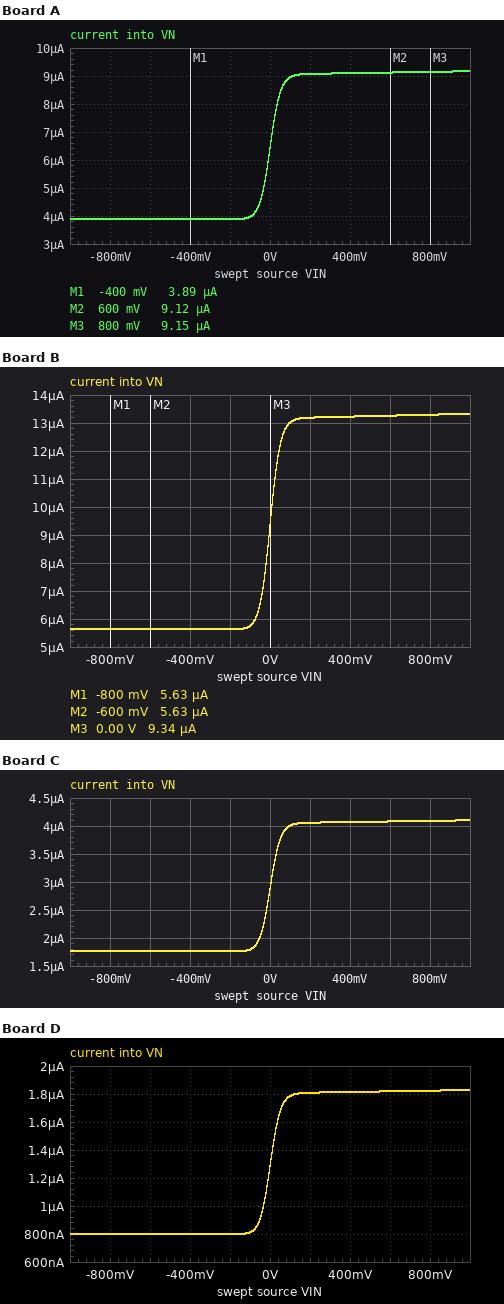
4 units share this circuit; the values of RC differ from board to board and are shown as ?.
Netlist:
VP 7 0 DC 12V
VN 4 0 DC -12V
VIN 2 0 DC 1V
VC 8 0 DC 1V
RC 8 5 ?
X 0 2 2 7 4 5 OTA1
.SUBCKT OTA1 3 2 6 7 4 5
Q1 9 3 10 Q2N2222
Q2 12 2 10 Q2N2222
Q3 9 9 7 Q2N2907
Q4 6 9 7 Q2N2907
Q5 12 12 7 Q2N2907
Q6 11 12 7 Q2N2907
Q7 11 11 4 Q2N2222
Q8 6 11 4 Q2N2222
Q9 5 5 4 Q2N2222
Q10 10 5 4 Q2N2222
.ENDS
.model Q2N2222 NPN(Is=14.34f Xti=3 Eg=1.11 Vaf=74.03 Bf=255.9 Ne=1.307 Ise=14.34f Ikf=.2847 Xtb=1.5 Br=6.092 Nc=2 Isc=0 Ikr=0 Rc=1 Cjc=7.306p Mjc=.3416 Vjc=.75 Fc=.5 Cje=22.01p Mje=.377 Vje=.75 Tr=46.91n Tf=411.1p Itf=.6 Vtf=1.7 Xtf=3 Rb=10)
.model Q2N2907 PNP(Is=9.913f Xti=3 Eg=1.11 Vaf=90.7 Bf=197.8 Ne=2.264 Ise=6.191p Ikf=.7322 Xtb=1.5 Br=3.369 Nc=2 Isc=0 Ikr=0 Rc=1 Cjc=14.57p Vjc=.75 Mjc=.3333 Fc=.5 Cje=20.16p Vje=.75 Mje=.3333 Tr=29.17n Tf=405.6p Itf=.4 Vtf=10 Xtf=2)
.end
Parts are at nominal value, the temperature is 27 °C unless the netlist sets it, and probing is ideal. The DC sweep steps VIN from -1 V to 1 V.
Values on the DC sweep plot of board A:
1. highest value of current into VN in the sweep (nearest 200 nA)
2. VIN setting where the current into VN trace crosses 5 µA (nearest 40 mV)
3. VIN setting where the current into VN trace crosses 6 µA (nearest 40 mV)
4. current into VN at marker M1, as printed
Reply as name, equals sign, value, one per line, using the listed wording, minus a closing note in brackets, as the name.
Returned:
highest value of current into VN in the sweep = 9.2 µA
VIN setting where the current into VN trace crosses 5 µA = -40 mV
VIN setting where the current into VN trace crosses 6 µA = 0 V
current into VN at marker M1, as printed = 3.89 µA
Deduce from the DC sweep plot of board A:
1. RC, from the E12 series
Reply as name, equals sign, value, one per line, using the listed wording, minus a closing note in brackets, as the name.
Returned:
RC, from the E12 series = 6.8 MΩ
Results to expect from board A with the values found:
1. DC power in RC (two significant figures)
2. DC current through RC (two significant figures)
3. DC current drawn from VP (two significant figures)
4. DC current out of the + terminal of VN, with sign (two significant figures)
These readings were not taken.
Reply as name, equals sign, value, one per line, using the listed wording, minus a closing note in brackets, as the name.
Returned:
DC power in RC = 23 µW
DC current through RC = 1.8 µA
DC current drawn from VP = 4.5 µA
DC current out of the + terminal of VN, with sign = -9.2 µA
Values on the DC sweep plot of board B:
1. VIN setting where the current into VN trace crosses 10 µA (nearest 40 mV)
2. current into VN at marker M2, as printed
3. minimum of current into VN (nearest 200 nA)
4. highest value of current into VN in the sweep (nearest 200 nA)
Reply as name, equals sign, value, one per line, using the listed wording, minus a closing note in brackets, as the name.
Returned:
VIN setting where the current into VN trace crosses 10 µA = 0 V
current into VN at marker M2, as printed = 5.63 µA
minimum of current into VN = 5.6 µA
highest value of current into VN in the sweep = 13.4 µA
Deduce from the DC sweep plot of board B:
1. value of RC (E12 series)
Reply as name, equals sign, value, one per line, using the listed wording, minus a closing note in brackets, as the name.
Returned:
value of RC = 4.7 MΩ
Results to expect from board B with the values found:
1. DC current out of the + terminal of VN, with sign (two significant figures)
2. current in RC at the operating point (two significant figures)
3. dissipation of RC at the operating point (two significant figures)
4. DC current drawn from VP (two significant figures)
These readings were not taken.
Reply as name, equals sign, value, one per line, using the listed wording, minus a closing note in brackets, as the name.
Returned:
DC current out of the + terminal of VN, with sign = -13 µA
current in RC at the operating point = 2.7 µA
dissipation of RC at the operating point = 33 µW
DC current drawn from VP = 6.6 µA
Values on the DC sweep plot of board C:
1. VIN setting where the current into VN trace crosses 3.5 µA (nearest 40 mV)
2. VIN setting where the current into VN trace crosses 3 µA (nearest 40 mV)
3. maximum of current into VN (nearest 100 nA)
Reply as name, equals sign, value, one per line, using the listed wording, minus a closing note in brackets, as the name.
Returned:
VIN setting where the current into VN trace crosses 3.5 µA = 40 mV
VIN setting where the current into VN trace crosses 3 µA = 0 V
maximum of current into VN = 4.1 µA
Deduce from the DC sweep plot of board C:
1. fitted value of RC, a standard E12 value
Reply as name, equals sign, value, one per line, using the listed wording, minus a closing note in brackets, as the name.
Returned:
fitted value of RC, a standard E12 value = 15 MΩ
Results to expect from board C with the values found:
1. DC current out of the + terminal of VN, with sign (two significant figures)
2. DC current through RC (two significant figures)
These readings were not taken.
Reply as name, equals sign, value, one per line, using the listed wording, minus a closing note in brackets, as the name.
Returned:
DC current out of the + terminal of VN, with sign = -4.1 µA
DC current through RC = 840 nA
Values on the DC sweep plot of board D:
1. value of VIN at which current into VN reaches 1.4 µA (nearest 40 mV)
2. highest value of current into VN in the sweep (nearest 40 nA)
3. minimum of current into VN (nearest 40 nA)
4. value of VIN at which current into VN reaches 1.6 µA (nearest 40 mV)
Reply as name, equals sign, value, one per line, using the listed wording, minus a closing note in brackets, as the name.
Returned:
value of VIN at which current into VN reaches 1.4 µA = 0 V
highest value of current into VN in the sweep = 1.84 µA
minimum of current into VN = 800 nA
value of VIN at which current into VN reaches 1.6 µA = 40 mV
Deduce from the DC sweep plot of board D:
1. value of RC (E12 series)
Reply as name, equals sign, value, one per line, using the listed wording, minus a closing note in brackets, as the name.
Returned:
value of RC = 33 MΩ
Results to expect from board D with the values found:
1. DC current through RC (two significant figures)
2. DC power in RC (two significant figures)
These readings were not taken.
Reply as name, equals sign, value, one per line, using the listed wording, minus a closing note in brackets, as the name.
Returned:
DC current through RC = 380 nA
DC power in RC = 4.8 µW
